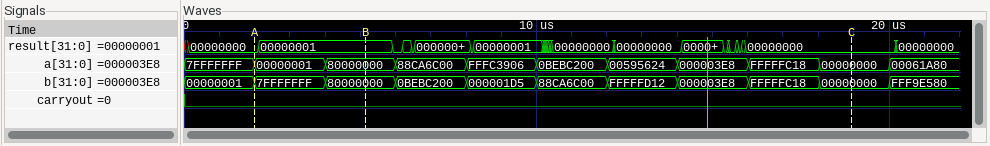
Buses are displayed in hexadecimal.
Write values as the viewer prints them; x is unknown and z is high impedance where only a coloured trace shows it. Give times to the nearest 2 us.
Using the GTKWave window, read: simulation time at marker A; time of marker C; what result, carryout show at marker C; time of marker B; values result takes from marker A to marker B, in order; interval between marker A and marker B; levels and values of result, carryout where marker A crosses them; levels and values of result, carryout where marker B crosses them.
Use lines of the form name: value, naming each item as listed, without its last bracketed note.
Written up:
simulation time at marker A: 2 us
time of marker C: 18 us
what result, carryout show at marker C: result=00000000, carryout=0
time of marker B: 6 us
values result takes from marker A to marker B, in order: 00000000, 00000001
interval between marker A and marker B: 4 us
levels and values of result, carryout where marker A crosses them: result=00000000, carryout=0
levels and values of result, carryout where marker B crosses them: result=00000001, carryout=0
